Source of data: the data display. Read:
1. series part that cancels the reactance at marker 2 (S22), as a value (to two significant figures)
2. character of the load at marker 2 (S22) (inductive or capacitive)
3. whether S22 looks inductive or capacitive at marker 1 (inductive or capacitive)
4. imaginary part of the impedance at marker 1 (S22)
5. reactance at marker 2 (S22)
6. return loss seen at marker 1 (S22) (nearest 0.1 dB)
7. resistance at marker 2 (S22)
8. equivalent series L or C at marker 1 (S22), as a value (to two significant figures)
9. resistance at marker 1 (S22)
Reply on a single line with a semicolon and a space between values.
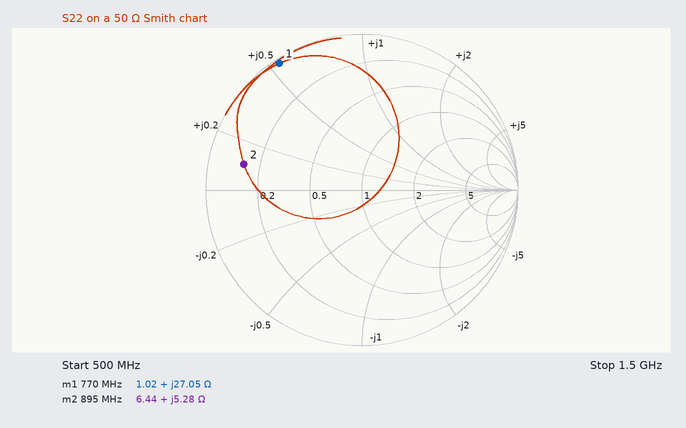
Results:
34 pF; inductive; inductive; +27.05 Ω; +5.28 Ω; 0.3 dB; 6.44 Ω; 5.6 nH; 1.02 Ω
